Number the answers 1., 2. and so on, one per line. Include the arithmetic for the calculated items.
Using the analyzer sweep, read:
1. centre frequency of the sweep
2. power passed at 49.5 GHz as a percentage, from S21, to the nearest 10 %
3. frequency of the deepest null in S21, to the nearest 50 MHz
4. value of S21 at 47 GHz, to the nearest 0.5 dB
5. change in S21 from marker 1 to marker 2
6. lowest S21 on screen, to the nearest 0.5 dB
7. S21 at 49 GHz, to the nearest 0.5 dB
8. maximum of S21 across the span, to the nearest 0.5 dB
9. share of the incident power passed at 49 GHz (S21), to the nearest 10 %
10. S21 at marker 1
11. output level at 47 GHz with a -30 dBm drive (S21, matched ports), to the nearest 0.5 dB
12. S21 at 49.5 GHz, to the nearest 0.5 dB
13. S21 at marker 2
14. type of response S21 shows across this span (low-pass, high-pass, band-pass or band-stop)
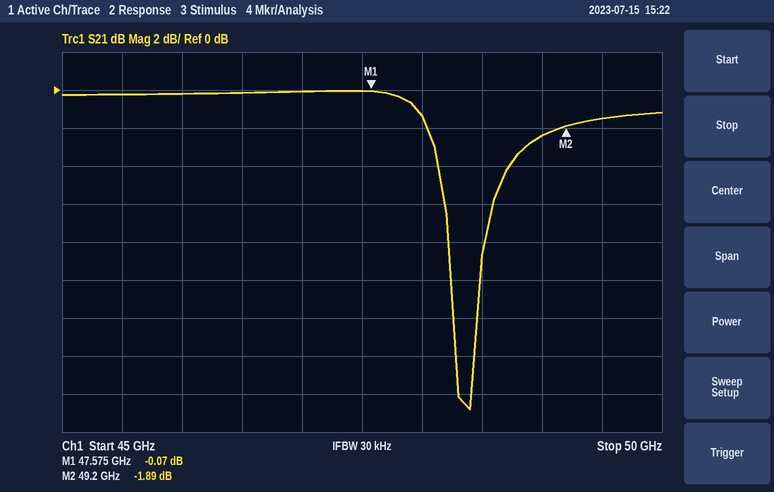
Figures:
1. 47.5 GHz
2. 10^(-1.5/10) ≈ 70.8 %, so 70 % to the nearest 10 %
3. 48.40 GHz
4. 0.0 dB
5. -1.89 − (-0.07) = -1.82 dB
6. -17.0 dB
7. -2.5 dB
8. 0.0 dB
9. 10^(-2.5/10) ≈ 56.2 %, so 60 % to the nearest 10 %
10. -0.07 dB
11. -30 dBm + (0.0 dB) = -30.0 dBm
12. -1.5 dB
13. -1.89 dB
14. band-stop
